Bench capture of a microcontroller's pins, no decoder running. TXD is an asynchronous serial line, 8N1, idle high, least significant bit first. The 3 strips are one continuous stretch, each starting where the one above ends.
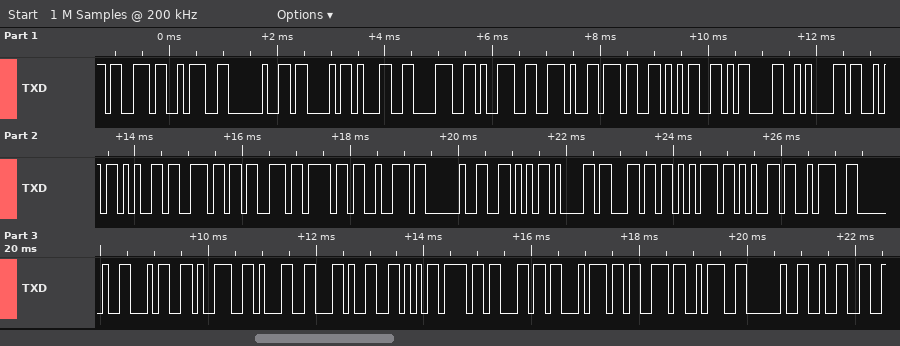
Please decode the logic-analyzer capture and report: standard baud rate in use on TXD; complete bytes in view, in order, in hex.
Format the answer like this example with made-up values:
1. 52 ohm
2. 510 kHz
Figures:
1. 9600 baud
2. 73 3A 20 43 31 38 39 2E 37 35 0D 0A 53 65 6E 73 6F 72 20 56 61 6C 75 65 3A 20 34 39 31 2C 56 6F 6C 74 73 3A 20 32
